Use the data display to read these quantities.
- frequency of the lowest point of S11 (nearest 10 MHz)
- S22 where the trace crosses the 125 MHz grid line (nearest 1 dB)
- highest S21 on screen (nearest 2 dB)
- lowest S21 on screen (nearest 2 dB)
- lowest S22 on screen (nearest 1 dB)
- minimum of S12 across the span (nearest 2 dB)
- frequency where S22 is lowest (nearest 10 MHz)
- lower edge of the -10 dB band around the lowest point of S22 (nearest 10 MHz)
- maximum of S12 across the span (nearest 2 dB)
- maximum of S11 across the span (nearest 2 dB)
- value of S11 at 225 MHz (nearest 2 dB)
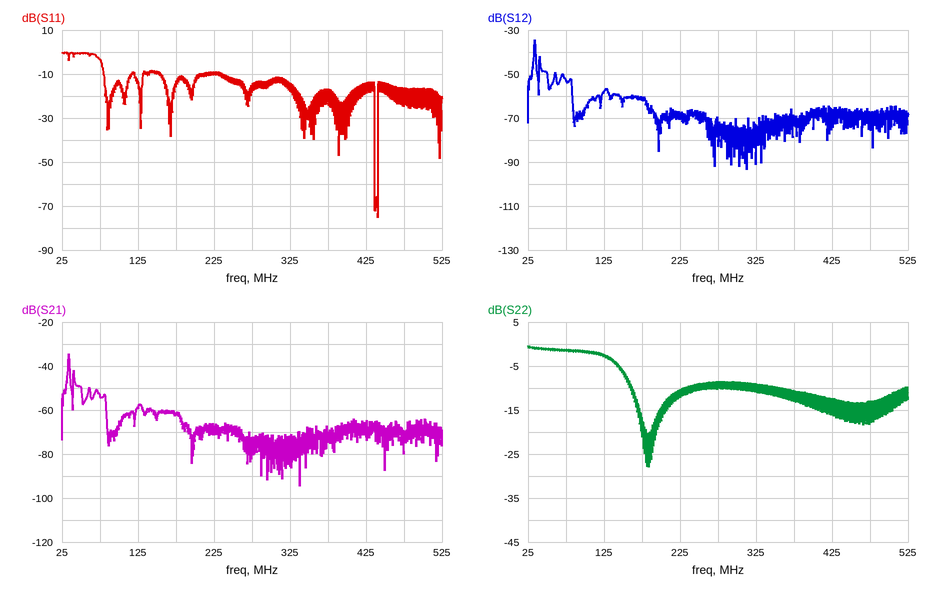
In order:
440 MHz
-3 dB
-34 dB
-94 dB
-28 dB
-94 dB
180 MHz
160 MHz
-34 dB
0 dB
-10 dB
